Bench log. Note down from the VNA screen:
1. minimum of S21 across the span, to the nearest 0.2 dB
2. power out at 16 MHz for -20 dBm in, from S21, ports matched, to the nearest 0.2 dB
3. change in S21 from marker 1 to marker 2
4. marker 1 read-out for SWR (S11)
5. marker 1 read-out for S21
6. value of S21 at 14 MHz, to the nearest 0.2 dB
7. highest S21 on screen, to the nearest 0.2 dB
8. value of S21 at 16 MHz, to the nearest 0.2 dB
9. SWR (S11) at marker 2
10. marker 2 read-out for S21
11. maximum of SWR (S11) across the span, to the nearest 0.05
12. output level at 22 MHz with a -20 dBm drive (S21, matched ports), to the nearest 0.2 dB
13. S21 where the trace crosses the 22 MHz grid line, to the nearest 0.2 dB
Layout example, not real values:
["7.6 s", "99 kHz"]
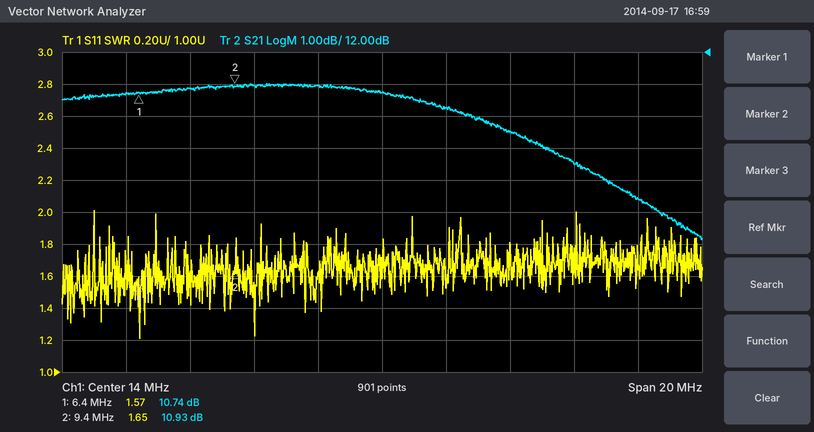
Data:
["6.2 dB", "-9.8 dBm", "0.19 dB", "1.57", "10.74 dB", "10.8 dB", "11.0 dB", "10.2 dB", "1.65", "10.93 dB", "2.00", "-12.6 dBm", "7.4 dB"]
